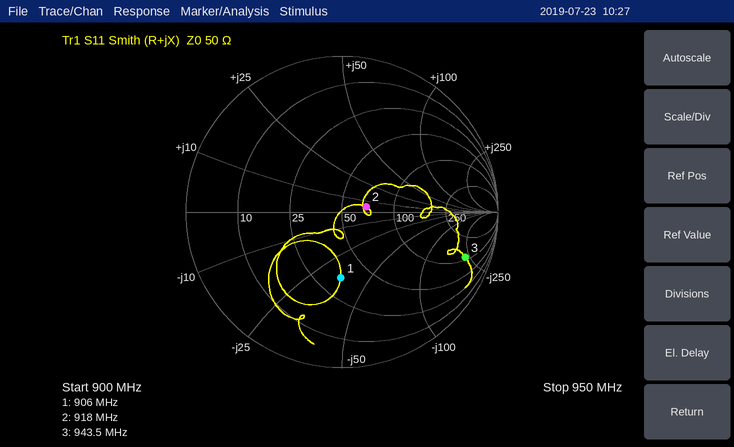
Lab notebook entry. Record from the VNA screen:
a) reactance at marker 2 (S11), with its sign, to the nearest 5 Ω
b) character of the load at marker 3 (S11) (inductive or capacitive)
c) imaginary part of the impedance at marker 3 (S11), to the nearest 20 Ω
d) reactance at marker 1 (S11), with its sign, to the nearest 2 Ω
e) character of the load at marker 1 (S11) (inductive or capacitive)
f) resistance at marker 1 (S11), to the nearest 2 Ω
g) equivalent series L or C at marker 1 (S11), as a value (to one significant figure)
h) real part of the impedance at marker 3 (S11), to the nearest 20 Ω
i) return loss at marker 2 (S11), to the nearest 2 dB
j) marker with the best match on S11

+5 Ω
capacitive
-220 Ω
-36 Ω
capacitive
34 Ω
5 pF
120 Ω
16 dB
marker 2
